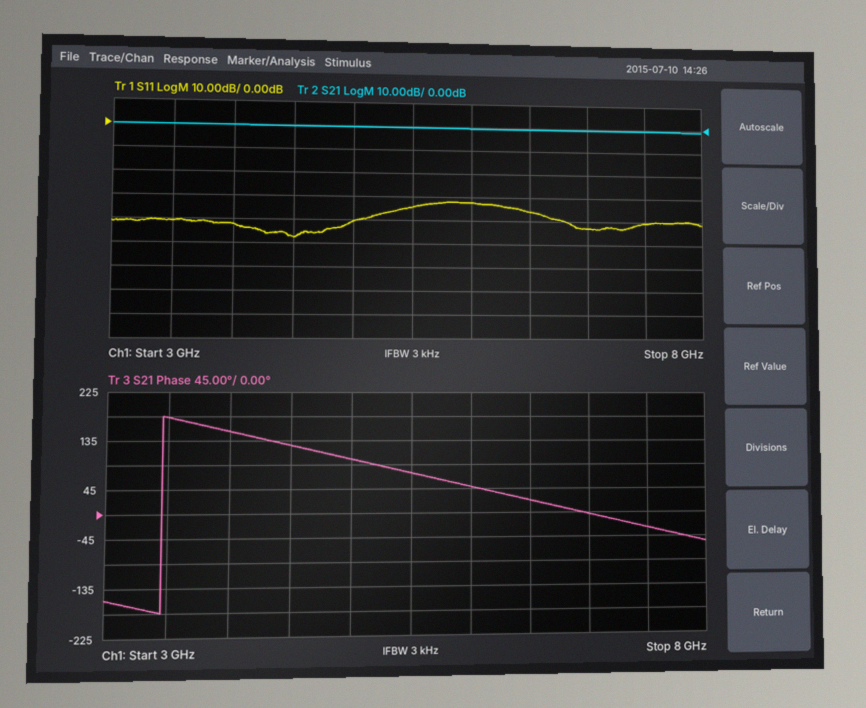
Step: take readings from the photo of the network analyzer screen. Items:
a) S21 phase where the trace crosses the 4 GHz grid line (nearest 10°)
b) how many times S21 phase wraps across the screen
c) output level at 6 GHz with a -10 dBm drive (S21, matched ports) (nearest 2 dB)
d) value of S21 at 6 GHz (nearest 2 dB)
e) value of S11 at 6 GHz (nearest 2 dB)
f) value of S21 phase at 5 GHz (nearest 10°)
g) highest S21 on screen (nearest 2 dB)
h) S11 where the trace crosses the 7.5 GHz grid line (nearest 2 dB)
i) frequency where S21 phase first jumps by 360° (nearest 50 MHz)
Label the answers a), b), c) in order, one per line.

a) 150°
b) 1
c) -10 dBm
d) 0 dB
e) -32 dB
f) 100°
g) 0 dB
h) -40 dB
i) 3.45 GHz
